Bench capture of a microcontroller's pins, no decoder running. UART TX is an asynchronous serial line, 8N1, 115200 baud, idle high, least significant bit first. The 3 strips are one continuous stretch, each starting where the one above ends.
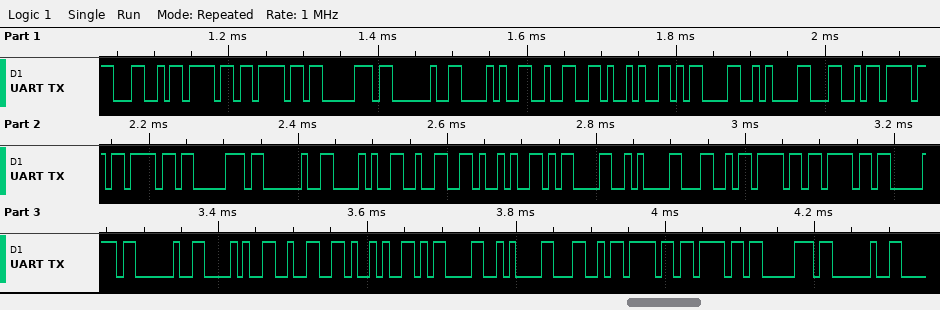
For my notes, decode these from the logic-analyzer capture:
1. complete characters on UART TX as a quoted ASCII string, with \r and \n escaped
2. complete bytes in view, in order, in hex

"Loop (2)\r\nLoop (2)\r\nLoop (2)\r\nLoop "
4C 6F 6F 70 20 28 32 29 0D 0A 4C 6F 6F 70 20 28 32 29 0D 0A 4C 6F 6F 70 20 28 32 29 0D 0A 4C 6F 6F 70 20
